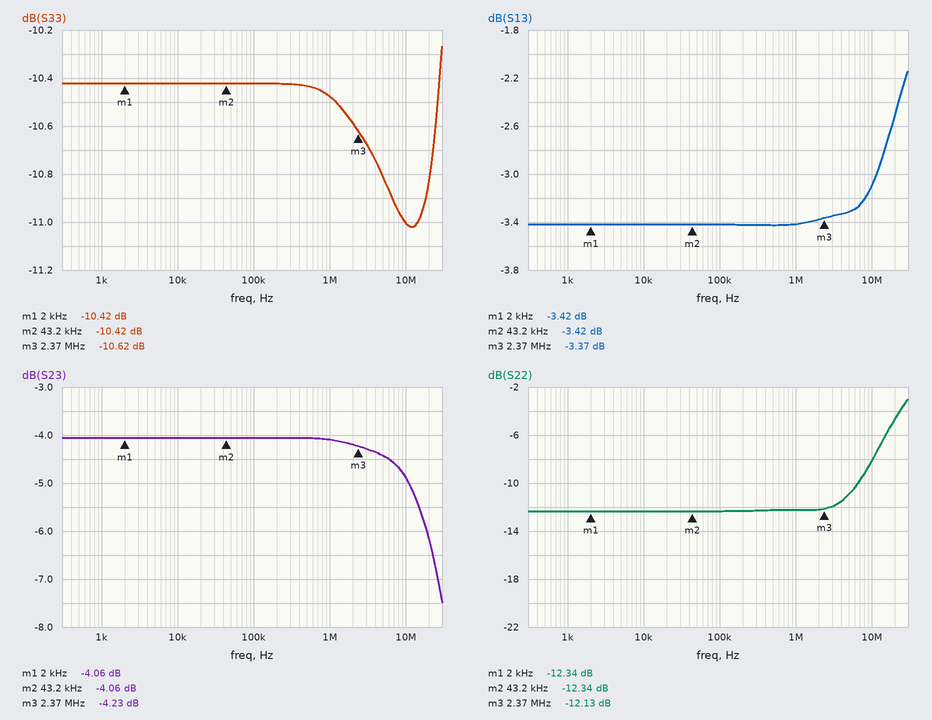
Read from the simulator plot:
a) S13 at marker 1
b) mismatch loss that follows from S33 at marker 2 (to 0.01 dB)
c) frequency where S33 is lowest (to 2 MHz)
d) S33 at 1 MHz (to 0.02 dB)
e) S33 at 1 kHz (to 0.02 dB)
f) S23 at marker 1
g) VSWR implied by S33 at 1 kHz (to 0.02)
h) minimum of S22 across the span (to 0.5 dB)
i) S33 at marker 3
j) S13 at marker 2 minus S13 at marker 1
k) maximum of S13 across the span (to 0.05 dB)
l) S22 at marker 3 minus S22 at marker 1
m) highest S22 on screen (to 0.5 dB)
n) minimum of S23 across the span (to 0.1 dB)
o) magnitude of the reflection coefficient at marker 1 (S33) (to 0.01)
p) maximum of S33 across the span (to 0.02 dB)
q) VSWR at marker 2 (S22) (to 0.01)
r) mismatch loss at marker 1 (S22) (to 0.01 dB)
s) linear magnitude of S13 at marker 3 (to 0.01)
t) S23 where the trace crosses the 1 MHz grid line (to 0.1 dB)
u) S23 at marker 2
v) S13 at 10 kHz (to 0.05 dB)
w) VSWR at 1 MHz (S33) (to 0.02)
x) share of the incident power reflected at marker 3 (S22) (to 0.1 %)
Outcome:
-3.42 dB
0.41 dB
12 MHz
-10.48 dB
-10.42 dB
-4.06 dB
1.86
-12.5 dB
-10.62 dB
0.00 dB
-2.15 dB
0.21 dB
-3.0 dB
-7.5 dB
0.30
-10.26 dB
1.64
0.26 dB
0.68
-4.1 dB
-4.06 dB
-3.40 dB
1.86
6.1 %
